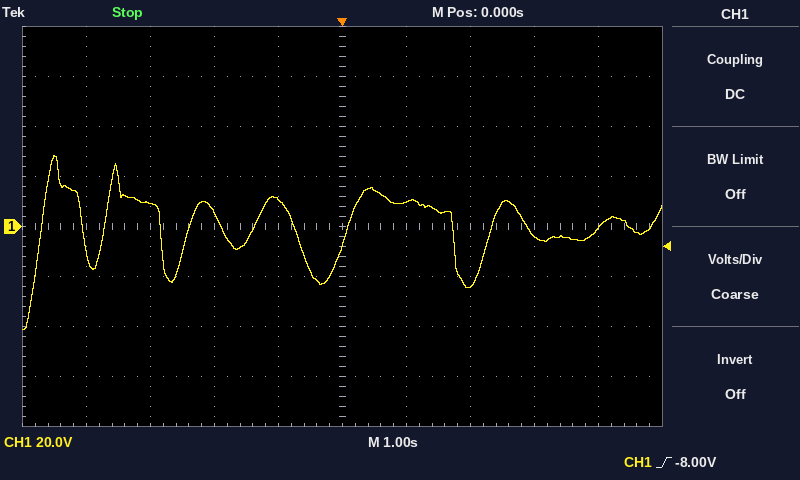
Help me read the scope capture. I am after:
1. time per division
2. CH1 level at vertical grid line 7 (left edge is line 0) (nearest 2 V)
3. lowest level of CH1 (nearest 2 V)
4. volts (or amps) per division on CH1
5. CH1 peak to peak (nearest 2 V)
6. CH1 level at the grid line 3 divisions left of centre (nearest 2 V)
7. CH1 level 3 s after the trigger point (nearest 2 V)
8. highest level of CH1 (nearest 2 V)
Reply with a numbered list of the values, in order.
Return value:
1. 1 s
2. -24 V
3. -42 V
4. 20 V
5. 70 V
6. 10 V
7. -4 V
8. 28 V
